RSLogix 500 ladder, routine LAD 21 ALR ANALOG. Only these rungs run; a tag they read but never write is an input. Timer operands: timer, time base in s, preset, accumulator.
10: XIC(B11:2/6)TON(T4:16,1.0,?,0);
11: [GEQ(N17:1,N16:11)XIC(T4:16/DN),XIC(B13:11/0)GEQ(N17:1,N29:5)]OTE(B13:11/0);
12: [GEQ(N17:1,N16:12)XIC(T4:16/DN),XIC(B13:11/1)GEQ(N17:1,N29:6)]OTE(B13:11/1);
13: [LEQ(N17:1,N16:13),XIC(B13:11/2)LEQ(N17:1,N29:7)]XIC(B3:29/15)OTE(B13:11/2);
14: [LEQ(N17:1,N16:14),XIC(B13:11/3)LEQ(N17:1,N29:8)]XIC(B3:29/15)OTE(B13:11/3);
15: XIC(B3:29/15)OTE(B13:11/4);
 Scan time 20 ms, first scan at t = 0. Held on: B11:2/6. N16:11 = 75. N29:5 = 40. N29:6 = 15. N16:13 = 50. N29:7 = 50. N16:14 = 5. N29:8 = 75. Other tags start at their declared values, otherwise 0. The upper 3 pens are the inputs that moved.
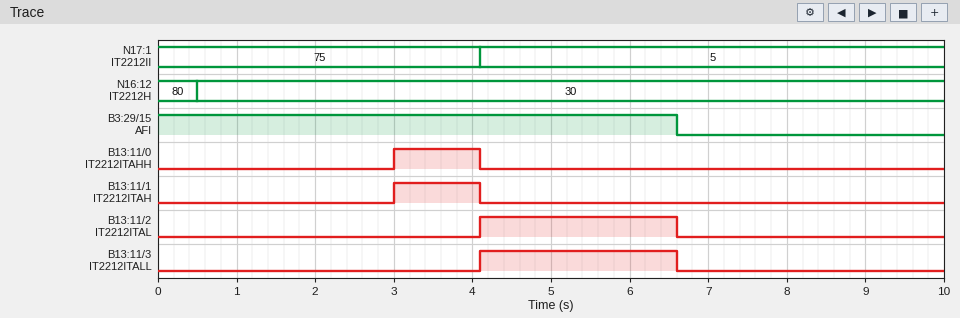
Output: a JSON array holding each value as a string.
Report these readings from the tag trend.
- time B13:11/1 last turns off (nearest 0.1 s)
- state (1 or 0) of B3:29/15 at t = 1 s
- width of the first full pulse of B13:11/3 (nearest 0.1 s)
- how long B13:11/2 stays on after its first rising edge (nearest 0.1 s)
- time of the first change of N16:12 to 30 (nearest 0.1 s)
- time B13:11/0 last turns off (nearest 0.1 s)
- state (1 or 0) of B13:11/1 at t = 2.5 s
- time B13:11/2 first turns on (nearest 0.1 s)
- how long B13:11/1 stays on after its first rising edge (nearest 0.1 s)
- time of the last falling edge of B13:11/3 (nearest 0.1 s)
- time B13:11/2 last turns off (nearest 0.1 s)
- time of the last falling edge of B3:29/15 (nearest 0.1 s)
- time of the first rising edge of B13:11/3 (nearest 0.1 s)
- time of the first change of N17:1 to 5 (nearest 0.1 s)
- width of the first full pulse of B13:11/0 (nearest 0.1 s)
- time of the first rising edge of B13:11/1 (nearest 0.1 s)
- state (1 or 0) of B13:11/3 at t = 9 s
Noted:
["4.1 s", "1", "2.5 s", "2.5 s", "0.5 s", "4.1 s", "0", "4.1 s", "1.1 s", "6.6 s", "6.6 s", "6.6 s", "4.1 s", "4.1 s", "1.1 s", "3.0 s", "0"]
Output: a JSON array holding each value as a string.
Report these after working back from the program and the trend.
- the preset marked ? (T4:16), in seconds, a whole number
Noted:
["3 s"]
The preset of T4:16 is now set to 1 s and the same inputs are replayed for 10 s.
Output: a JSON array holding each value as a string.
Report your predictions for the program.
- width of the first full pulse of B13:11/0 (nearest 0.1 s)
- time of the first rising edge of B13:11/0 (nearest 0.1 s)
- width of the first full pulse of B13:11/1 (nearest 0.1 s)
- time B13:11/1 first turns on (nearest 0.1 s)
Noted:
["3.1 s", "1.0 s", "3.1 s", "1.0 s"]
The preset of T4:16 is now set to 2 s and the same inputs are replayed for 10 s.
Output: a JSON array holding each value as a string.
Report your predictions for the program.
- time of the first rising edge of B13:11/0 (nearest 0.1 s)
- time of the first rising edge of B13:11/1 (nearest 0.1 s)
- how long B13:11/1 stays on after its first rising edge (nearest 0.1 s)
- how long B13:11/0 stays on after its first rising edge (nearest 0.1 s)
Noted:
["2.0 s", "2.0 s", "2.1 s", "2.1 s"]
